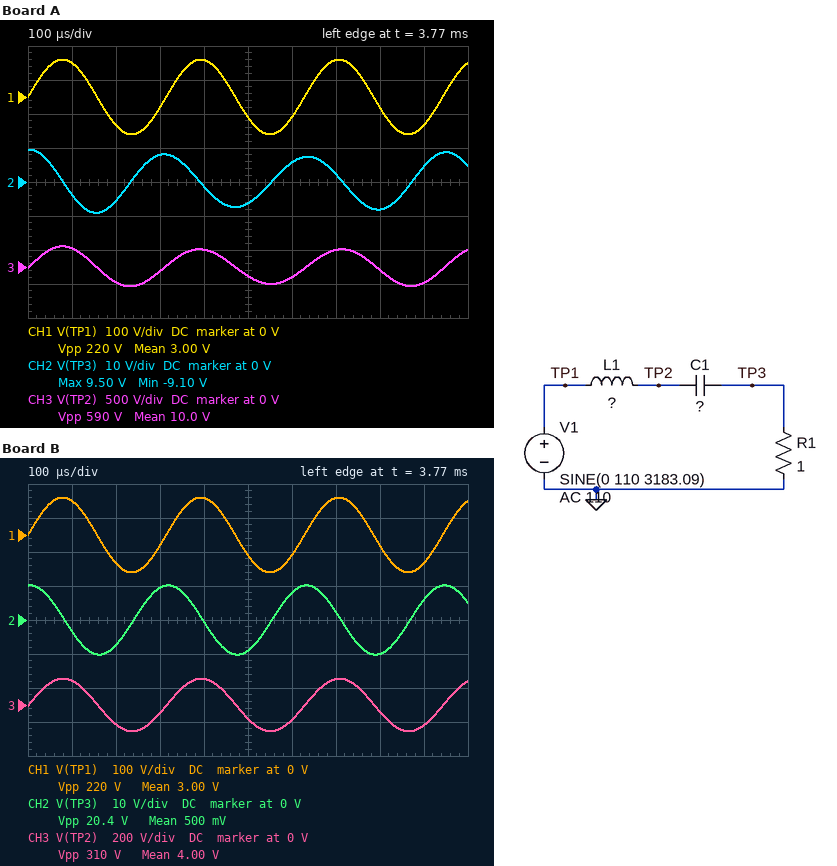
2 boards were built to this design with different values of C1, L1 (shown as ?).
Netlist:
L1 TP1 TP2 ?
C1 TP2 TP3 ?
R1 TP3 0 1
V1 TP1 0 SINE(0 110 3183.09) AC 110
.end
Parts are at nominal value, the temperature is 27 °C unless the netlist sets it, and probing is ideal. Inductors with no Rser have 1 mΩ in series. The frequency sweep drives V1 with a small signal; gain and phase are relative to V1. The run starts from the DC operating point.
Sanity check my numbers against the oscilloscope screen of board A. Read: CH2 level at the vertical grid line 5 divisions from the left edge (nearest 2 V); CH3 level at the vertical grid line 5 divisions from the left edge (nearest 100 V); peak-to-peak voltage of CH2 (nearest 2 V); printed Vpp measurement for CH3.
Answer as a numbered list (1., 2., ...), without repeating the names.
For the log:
1. -6 V
2. -100 V
3. 18 V
4. 590 V
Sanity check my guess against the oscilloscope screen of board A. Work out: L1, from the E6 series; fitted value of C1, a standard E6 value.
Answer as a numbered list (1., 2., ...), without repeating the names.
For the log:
1. 1 mH
2. 1.5 µF
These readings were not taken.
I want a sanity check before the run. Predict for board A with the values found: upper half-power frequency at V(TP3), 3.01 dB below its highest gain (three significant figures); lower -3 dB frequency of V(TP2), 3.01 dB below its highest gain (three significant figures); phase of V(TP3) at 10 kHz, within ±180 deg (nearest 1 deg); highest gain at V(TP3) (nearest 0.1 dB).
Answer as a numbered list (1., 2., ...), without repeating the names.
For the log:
1. 4.19 kHz
2. 4.03 kHz
3. -89 deg
4. 0 dB
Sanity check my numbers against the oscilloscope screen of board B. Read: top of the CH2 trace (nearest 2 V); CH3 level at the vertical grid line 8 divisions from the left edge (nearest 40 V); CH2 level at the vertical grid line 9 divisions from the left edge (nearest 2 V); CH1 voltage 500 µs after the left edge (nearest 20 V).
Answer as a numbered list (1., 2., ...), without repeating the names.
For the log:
1. 10 V
2. -40 V
3. 6 V
4. -60 V
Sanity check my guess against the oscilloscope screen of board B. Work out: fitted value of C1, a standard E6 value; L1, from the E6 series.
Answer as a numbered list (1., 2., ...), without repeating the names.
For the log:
1. 3.3 µF
2. 220 µH
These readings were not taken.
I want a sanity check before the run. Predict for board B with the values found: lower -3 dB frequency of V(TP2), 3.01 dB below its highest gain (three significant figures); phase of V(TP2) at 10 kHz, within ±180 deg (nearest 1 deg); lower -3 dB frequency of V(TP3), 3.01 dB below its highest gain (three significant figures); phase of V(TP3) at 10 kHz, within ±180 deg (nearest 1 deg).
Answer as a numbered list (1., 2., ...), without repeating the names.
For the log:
1. 5.51 kHz
2. -162 deg
3. 5.56 kHz
4. -84 deg
